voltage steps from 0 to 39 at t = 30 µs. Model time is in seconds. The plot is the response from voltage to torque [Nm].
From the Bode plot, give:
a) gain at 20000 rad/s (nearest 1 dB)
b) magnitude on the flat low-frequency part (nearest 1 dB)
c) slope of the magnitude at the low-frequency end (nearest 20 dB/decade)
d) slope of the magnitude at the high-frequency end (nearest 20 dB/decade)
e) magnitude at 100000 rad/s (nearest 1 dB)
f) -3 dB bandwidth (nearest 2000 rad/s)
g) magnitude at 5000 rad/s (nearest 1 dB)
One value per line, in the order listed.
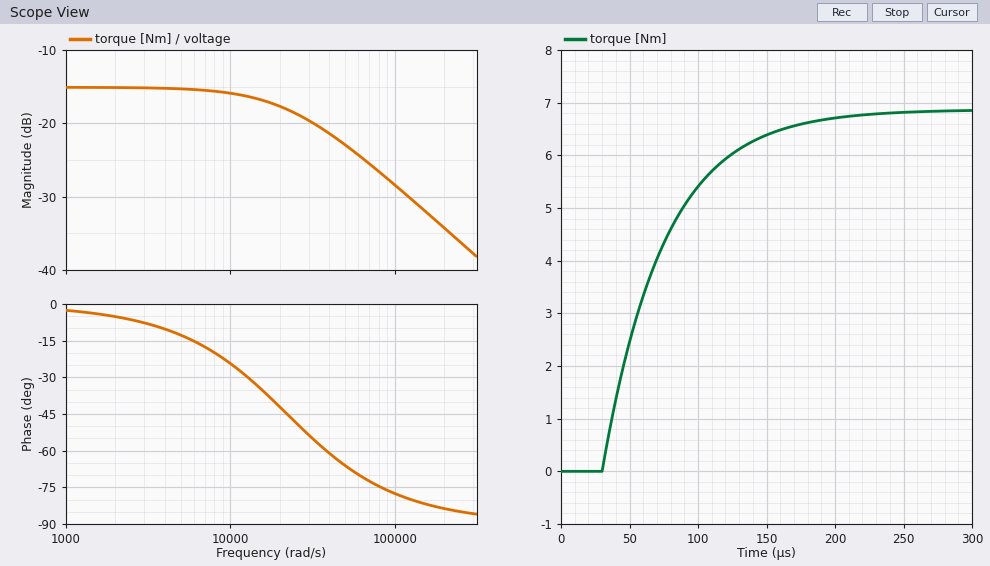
-18 dB
-15 dB
0 dB/decade
-20 dB/decade
-28 dB
22000 rad/s
-15 dB
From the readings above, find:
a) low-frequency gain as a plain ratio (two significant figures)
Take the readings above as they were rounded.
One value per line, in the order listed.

0.18
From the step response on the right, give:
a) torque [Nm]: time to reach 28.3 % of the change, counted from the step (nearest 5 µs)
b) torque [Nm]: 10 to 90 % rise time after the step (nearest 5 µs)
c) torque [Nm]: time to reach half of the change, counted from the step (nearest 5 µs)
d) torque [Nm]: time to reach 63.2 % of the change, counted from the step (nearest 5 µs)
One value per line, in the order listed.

15 µs
100 µs
30 µs
45 µs
